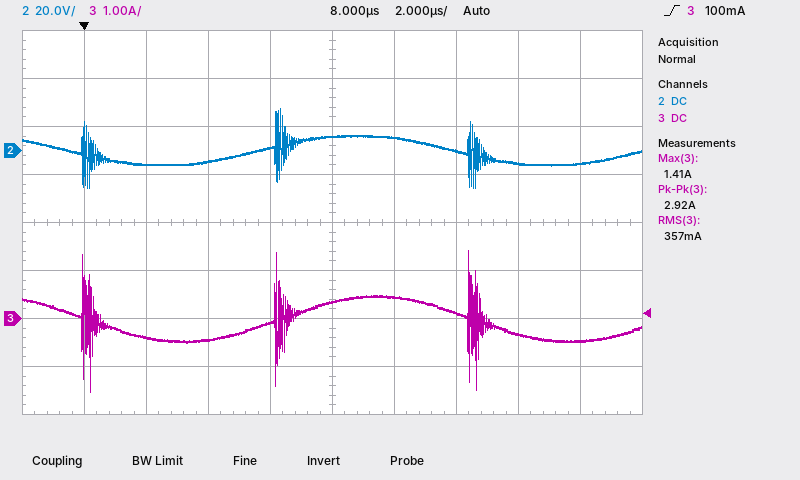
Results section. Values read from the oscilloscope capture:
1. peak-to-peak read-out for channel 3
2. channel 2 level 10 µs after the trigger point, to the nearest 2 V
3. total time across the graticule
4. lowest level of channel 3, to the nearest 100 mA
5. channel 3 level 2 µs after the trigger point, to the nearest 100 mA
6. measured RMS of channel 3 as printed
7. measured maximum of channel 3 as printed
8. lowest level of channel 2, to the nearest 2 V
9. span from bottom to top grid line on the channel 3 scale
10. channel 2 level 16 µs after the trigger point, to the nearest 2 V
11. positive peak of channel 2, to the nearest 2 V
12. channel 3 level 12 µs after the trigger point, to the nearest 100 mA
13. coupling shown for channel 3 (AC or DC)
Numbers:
2.92 A
6 V
20 µs
-1.5 A
-400 mA
357 mA
1.41 A
-16 V
8 A
-6 V
18 V
100 mA
DC
